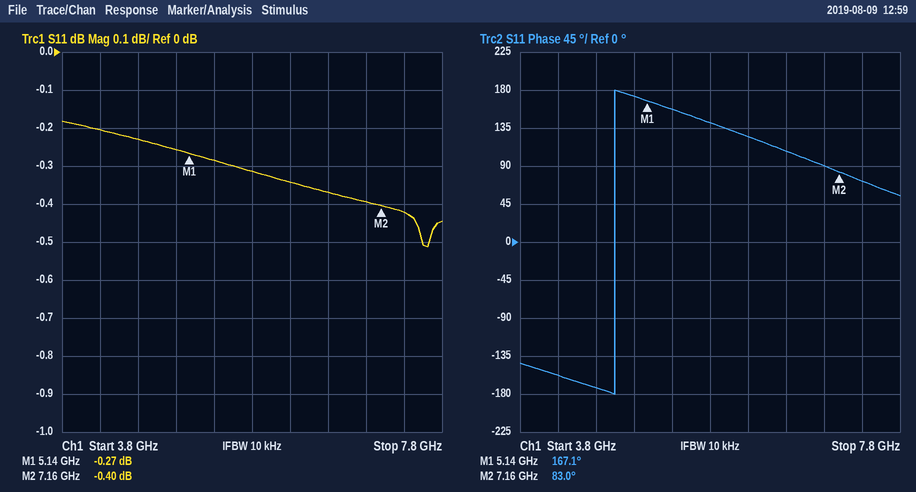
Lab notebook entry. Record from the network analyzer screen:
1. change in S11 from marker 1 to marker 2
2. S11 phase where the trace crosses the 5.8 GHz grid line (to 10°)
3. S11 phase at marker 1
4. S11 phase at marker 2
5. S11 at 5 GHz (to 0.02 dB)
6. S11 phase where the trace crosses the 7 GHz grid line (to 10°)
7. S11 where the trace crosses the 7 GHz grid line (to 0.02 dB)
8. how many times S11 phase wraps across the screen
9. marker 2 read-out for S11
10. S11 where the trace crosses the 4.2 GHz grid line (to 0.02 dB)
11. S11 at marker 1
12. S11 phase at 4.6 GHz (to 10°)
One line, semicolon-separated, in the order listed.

-0.13 dB; 140°; 167.1°; 83.0°; -0.26 dB; 90°; -0.40 dB; 1; -0.40 dB; -0.20 dB; -0.27 dB; -170°
